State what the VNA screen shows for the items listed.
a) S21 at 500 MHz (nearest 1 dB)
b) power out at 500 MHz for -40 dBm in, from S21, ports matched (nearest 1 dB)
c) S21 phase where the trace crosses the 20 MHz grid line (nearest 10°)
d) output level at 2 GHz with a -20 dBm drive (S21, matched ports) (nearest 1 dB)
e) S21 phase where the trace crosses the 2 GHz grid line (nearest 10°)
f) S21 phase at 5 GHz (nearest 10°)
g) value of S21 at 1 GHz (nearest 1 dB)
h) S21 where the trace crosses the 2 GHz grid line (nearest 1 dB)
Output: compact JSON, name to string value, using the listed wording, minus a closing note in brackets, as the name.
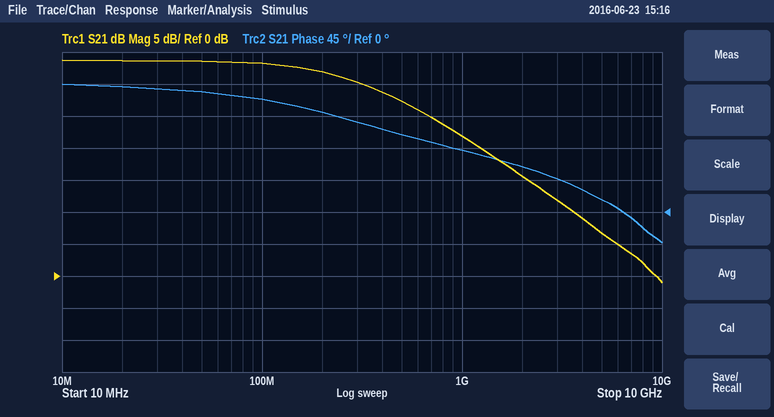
{"S21 at 500 MHz": "27 dB", "power out at 500 MHz for -40 dBm in, from S21, ports matched": "-13 dBm", "S21 phase where the trace crosses the 20 MHz grid line": "180°", "output level at 2 GHz with a -20 dBm drive (S21, matched ports)": "-4 dBm", "S21 phase where the trace crosses the 2 GHz grid line": "60°", "S21 phase at 5 GHz": "20°", "value of S21 at 1 GHz": "22 dB", "S21 where the trace crosses the 2 GHz grid line": "16 dB"}
